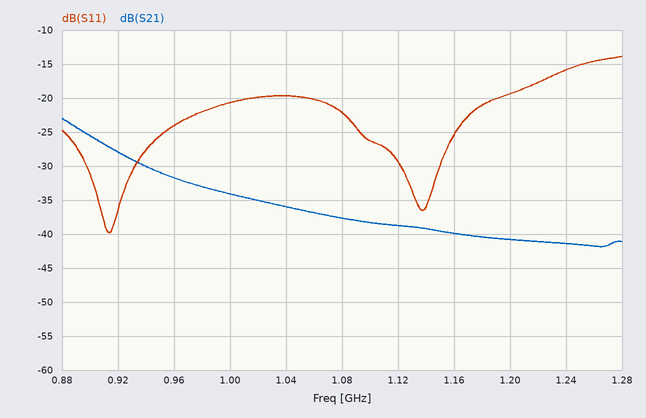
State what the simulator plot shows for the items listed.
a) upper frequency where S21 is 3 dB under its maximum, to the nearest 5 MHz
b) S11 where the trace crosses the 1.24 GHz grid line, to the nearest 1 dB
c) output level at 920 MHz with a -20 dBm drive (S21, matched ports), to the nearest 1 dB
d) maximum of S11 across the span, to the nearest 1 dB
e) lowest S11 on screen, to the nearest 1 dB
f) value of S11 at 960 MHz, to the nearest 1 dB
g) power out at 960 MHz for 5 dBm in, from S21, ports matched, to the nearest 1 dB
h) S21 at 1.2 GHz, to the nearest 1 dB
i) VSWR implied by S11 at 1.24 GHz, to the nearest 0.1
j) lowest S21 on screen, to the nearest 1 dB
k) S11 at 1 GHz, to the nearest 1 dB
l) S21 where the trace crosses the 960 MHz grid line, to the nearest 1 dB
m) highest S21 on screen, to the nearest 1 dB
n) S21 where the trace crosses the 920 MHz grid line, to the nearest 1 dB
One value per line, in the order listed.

905 MHz
-16 dB
-48 dBm
-14 dB
-40 dB
-24 dB
-27 dBm
-41 dB
1.4
-42 dB
-21 dB
-32 dB
-23 dB
-28 dB
